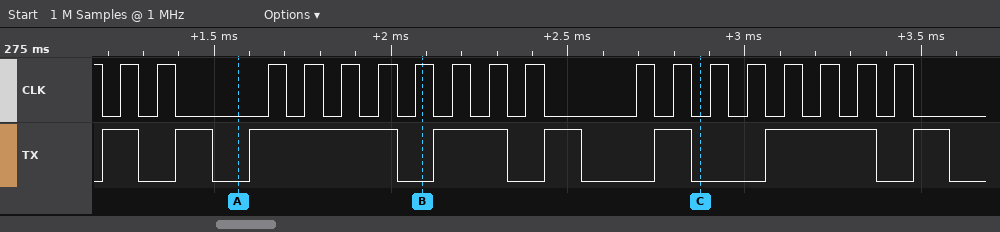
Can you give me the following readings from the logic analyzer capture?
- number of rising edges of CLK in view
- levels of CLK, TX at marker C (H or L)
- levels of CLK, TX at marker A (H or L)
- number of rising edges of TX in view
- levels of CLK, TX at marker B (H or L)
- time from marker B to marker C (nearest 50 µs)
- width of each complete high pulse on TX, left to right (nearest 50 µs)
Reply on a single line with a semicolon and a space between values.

18; CLK=L, TX=L; CLK=L, TX=L; 8; CLK=H, TX=L; 800 µs; 100 µs, 100 µs, 400 µs, 200 µs, 100 µs, 100 µs, 300 µs, 100 µs
